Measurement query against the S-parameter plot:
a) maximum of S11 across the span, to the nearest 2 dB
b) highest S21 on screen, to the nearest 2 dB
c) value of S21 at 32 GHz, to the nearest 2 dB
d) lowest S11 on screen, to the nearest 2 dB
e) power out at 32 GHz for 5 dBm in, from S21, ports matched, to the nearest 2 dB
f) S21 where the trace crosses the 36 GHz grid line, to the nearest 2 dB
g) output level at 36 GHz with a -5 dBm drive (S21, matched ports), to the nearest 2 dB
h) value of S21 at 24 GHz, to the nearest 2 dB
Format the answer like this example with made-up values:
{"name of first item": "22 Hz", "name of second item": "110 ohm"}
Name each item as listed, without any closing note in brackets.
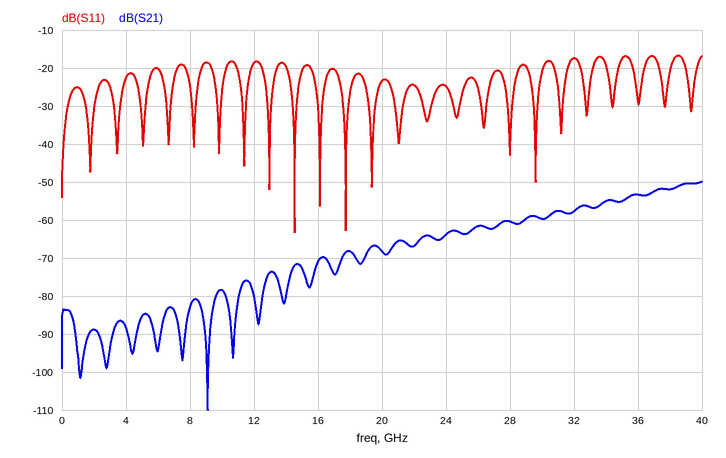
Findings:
{"maximum of S11 across the span, to the nearest 2 dB": "-16 dB", "highest S21 on screen, to the nearest 2 dB": "-50 dB", "value of S21 at 32 GHz, to the nearest 2 dB": "-58 dB", "lowest S11 on screen, to the nearest 2 dB": "-64 dB", "power out at 32 GHz for 5 dBm in, from S21, ports matched, to the nearest 2 dB": "-52 dBm", "S21 where the trace crosses the 36 GHz grid line, to the nearest 2 dB": "-54 dB", "output level at 36 GHz with a -5 dBm drive (S21, matched ports), to the nearest 2 dB": "-58 dBm", "value of S21 at 24 GHz, to the nearest 2 dB": "-64 dB"}
